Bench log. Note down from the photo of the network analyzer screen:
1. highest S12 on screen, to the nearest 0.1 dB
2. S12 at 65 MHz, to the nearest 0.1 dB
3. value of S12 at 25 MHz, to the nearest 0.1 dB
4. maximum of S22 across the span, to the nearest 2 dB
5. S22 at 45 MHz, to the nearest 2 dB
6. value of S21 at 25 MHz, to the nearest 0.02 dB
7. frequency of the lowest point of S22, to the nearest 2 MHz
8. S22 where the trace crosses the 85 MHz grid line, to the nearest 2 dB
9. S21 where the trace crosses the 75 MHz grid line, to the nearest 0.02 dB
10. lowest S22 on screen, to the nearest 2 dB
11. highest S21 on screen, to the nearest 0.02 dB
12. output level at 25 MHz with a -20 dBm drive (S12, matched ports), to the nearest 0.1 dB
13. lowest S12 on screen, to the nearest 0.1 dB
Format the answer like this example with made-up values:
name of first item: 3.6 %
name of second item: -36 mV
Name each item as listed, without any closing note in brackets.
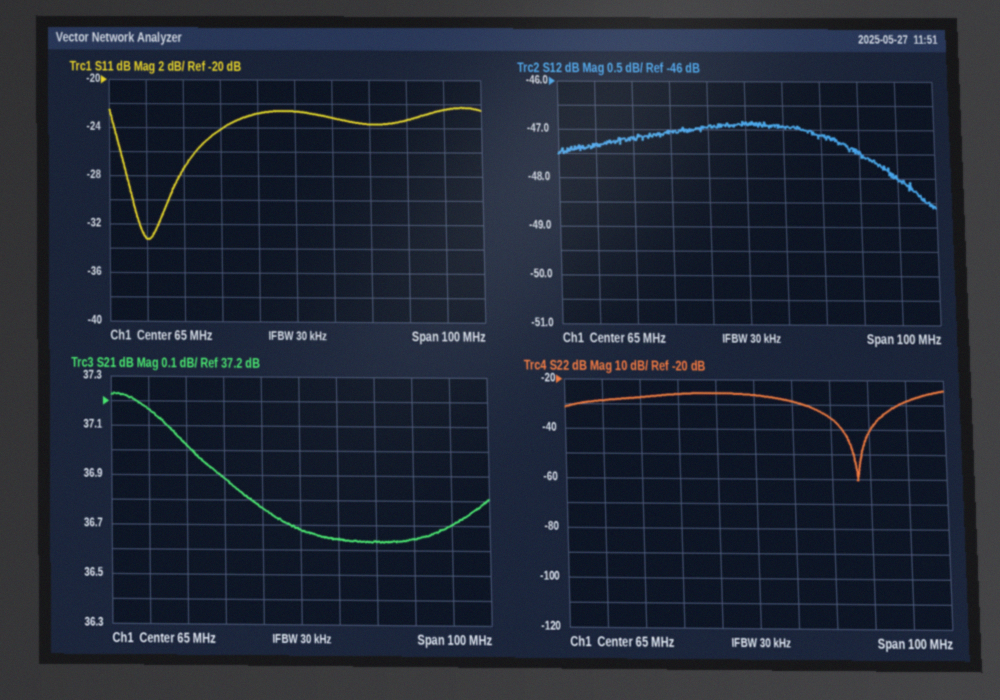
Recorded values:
highest S12 on screen, to the nearest 0.1 dB: -46.8 dB
S12 at 65 MHz, to the nearest 0.1 dB: -46.9 dB
value of S12 at 25 MHz, to the nearest 0.1 dB: -47.3 dB
maximum of S22 across the span, to the nearest 2 dB: -24 dB
S22 at 45 MHz, to the nearest 2 dB: -26 dB
value of S21 at 25 MHz, to the nearest 0.02 dB: 37.16 dB
frequency of the lowest point of S22, to the nearest 2 MHz: 92 MHz
S22 where the trace crosses the 85 MHz grid line, to the nearest 2 dB: -36 dB
S21 where the trace crosses the 75 MHz grid line, to the nearest 0.02 dB: 36.64 dB
lowest S22 on screen, to the nearest 2 dB: -60 dB
highest S21 on screen, to the nearest 0.02 dB: 37.24 dB
output level at 25 MHz with a -20 dBm drive (S12, matched ports), to the nearest 0.1 dB: -67.3 dBm
lowest S12 on screen, to the nearest 0.1 dB: -48.6 dB
